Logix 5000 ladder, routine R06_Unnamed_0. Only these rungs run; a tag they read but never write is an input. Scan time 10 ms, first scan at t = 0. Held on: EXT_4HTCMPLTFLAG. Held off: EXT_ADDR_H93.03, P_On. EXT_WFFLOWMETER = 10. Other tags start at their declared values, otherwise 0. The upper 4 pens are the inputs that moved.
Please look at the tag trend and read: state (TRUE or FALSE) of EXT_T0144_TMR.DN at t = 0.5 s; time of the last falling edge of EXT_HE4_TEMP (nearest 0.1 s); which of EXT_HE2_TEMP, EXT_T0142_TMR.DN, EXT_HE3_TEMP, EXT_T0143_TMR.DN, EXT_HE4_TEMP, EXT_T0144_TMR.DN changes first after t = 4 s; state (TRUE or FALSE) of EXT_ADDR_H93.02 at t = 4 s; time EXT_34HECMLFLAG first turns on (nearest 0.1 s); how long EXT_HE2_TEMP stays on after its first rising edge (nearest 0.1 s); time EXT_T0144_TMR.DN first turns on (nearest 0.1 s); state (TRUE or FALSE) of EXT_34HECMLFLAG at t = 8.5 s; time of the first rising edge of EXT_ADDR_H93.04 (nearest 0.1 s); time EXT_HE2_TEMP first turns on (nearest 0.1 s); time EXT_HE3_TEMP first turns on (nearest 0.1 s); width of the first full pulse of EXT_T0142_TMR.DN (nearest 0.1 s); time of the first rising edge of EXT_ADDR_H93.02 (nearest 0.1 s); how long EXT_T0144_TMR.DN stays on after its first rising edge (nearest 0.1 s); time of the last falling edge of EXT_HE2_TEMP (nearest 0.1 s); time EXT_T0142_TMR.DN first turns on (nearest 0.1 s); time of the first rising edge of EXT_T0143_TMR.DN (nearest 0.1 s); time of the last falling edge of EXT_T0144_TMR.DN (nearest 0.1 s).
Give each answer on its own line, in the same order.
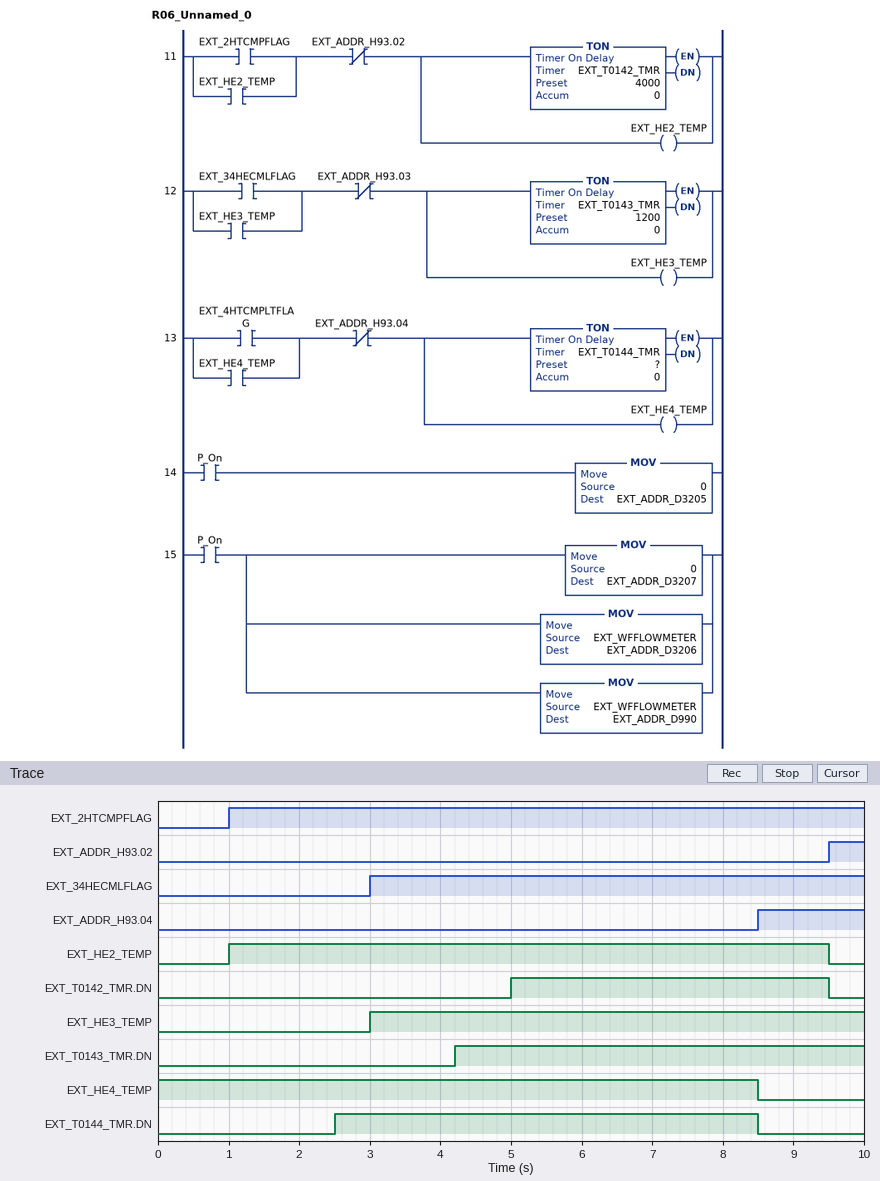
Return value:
FALSE
8.5 s
EXT_T0143_TMR.DN
FALSE
3.0 s
8.5 s
2.5 s
TRUE
8.5 s
1.0 s
3.0 s
4.5 s
9.5 s
6.0 s
9.5 s
5.0 s
4.2 s
8.5 s
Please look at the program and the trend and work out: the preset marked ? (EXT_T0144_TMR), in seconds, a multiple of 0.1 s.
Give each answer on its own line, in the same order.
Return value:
2.5 s
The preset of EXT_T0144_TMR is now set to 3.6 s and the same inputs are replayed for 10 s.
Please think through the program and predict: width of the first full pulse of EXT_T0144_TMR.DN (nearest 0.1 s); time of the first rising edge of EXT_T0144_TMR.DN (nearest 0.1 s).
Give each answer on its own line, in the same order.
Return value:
4.9 s
3.6 s
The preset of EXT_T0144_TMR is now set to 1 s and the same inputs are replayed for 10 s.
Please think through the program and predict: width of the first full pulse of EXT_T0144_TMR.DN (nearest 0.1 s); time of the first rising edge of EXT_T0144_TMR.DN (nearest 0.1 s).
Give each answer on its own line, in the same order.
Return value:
7.5 s
1.0 s
